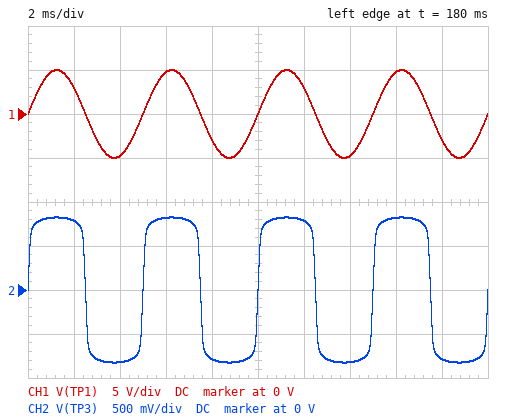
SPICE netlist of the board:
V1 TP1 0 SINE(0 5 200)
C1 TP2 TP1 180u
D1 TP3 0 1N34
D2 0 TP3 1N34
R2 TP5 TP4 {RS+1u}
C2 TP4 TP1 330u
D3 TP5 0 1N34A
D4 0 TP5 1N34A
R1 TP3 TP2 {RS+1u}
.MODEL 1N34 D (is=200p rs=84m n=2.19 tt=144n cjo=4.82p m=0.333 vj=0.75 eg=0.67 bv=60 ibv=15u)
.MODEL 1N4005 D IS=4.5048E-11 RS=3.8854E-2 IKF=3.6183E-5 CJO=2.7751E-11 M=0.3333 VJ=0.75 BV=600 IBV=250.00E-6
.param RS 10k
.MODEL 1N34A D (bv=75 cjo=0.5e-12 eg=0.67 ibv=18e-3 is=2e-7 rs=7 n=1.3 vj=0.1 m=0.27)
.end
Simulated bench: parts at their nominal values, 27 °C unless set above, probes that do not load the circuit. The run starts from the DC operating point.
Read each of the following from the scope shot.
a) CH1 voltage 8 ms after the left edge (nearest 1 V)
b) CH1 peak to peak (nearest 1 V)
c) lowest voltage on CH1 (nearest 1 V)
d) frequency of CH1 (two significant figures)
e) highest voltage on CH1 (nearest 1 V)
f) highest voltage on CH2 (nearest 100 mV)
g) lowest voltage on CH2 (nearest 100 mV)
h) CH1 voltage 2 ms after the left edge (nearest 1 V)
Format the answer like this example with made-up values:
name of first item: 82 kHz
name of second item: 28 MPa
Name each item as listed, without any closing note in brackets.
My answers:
CH1 voltage 8 ms after the left edge: -3 V
CH1 peak to peak: 10 V
lowest voltage on CH1: -5 V
frequency of CH1: 200 Hz
highest voltage on CH1: 5 V
highest voltage on CH2: 800 mV
lowest voltage on CH2: -800 mV
CH1 voltage 2 ms after the left edge: 3 V
